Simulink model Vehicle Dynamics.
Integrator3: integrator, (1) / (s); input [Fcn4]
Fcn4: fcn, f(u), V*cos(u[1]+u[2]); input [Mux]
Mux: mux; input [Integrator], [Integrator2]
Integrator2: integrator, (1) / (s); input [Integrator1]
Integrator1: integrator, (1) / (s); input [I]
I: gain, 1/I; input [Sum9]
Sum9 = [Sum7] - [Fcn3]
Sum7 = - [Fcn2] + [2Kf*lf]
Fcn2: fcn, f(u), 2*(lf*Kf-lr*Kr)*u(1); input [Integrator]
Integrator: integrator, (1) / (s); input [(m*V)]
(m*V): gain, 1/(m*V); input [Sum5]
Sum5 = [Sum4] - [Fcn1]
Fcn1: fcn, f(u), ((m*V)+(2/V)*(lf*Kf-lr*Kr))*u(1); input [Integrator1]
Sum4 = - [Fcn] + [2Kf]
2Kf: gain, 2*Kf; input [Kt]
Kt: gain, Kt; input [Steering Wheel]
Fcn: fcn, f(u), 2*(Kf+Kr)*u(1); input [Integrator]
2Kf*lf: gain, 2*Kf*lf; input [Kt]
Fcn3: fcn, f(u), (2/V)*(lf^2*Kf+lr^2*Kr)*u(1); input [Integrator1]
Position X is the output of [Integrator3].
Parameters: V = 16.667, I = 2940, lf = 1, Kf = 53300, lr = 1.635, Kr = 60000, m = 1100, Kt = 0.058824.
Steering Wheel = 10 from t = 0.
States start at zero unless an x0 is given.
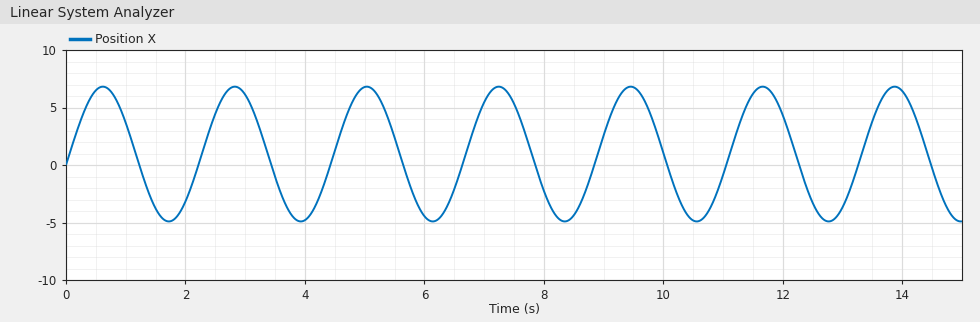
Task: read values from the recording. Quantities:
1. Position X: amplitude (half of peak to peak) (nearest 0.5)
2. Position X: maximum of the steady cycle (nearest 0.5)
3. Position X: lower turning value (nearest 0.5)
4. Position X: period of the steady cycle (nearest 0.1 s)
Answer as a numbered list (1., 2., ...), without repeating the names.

1. 6.0
2. 7.0
3. -5.0
4. 2.2 s
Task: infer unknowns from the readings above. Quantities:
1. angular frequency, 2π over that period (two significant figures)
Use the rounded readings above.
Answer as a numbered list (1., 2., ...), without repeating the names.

1. 2.9 rad/s
